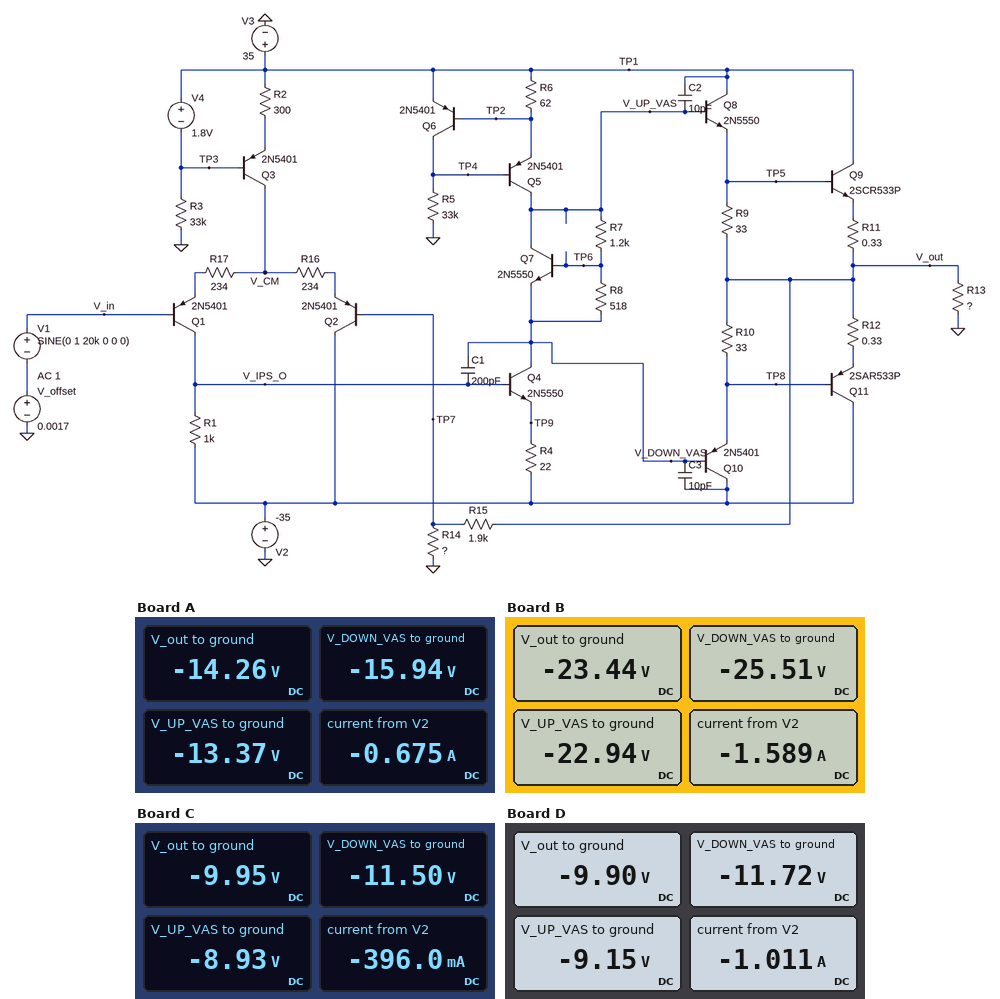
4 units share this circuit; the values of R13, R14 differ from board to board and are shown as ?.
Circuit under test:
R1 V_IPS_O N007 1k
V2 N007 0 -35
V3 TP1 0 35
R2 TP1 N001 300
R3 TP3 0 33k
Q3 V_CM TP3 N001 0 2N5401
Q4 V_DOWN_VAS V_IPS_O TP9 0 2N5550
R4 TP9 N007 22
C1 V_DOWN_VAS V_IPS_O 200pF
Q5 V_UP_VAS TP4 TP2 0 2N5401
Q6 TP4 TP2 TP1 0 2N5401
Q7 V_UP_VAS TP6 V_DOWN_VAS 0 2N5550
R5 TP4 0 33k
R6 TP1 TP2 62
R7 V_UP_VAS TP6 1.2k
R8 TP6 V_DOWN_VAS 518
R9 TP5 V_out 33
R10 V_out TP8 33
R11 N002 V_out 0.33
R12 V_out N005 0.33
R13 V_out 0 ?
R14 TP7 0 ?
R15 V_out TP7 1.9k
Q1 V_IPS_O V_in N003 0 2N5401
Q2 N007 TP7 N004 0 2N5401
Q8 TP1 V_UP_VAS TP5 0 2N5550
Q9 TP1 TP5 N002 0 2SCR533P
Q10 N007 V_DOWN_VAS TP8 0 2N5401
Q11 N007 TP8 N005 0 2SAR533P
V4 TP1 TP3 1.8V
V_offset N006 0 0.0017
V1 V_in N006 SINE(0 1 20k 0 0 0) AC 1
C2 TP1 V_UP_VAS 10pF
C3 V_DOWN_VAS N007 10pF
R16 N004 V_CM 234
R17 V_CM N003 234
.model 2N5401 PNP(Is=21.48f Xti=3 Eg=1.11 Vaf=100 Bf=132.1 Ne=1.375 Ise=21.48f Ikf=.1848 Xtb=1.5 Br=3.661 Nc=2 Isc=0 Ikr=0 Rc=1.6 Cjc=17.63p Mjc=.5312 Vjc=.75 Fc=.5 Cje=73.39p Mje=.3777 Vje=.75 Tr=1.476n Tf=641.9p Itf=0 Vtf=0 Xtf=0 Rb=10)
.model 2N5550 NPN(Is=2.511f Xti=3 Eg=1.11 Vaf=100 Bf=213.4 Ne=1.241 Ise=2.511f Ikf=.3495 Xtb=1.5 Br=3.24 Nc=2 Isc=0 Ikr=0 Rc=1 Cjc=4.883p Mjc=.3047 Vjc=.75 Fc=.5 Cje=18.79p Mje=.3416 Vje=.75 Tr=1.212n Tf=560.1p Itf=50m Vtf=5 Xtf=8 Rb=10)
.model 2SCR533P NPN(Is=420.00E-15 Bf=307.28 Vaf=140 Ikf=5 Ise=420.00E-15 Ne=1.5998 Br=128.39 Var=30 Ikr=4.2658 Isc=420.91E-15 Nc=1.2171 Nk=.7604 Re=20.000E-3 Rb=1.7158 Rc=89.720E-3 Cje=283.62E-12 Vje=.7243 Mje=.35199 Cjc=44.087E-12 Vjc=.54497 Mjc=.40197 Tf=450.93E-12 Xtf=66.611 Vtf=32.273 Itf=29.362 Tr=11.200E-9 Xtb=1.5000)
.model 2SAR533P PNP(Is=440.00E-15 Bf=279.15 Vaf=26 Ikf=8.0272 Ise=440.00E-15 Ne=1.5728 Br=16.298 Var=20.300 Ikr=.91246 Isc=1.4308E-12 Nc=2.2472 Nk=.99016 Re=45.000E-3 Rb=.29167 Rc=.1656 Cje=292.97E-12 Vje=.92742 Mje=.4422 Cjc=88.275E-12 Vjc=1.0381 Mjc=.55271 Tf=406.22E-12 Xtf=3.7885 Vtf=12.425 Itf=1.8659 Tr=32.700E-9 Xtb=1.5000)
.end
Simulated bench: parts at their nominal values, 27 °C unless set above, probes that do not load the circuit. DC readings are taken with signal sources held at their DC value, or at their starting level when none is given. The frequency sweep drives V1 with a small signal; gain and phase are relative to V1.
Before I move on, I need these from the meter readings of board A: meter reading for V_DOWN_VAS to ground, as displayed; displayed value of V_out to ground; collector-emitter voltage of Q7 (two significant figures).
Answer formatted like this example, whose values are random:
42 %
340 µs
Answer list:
-15.94 V
-14.26 V
2.6 V
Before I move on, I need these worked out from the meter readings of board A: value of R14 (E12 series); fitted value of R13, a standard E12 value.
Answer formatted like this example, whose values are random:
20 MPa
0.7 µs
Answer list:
56 Ω
22 Ω
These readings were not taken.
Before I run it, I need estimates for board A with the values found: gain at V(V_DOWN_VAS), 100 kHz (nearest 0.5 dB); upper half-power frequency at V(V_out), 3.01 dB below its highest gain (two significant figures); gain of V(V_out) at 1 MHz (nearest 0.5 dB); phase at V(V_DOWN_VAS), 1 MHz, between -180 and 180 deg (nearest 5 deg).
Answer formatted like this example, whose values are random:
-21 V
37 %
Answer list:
23.0 dB
43 kHz
3.5 dB
-90 deg
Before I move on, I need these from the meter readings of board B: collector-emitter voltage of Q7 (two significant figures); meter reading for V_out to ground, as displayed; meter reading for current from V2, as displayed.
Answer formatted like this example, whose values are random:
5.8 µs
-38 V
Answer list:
2.6 V
-23.44 V
-1.589 A
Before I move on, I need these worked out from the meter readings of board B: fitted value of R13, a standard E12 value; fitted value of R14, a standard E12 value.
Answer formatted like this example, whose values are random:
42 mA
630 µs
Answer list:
15 Ω
33 Ω
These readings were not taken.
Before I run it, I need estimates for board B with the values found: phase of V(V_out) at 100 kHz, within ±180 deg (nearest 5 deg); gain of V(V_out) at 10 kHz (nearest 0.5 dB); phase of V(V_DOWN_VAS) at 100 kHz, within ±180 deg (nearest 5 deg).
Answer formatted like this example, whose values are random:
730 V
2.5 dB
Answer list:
-75 deg
34.5 dB
-75 deg
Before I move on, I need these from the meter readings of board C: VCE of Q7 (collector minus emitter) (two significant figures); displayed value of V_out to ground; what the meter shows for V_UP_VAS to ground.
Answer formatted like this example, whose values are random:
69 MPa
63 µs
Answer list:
2.6 V
-9.95 V
-8.93 V
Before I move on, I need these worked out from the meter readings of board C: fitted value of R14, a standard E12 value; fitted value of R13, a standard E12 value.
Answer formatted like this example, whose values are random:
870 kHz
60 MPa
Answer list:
82 Ω
27 Ω
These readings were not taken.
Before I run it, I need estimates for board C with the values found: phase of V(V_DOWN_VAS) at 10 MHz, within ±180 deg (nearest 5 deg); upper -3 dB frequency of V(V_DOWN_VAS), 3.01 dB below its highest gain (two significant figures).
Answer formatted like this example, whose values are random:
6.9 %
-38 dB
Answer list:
-130 deg
62 kHz
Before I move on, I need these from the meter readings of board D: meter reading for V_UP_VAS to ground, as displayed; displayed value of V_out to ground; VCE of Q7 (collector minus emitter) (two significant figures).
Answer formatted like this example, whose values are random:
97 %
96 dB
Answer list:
-9.15 V
-9.90 V
2.6 V
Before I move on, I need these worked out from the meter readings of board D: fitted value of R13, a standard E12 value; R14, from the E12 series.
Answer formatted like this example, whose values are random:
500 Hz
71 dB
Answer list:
10 Ω
82 Ω
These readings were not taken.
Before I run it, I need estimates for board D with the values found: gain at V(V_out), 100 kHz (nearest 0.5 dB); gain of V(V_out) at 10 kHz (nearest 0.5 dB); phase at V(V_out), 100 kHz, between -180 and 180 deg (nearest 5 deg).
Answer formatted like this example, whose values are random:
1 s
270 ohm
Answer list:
22.0 dB
27.5 dB
-60 deg
